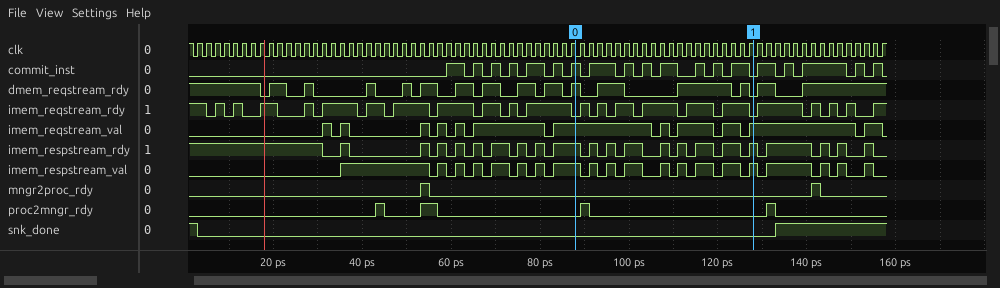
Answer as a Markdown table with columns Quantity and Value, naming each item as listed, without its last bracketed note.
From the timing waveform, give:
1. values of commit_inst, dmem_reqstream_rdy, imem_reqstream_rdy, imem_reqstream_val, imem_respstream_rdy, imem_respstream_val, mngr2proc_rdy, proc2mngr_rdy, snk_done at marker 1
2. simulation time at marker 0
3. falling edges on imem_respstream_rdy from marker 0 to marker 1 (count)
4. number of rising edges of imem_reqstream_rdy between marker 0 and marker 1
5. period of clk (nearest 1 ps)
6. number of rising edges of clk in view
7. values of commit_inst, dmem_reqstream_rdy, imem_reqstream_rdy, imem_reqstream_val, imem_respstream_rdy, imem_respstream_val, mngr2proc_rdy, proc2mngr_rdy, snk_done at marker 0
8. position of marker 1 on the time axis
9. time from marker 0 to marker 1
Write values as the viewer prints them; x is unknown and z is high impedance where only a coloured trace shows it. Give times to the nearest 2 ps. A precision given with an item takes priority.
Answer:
| Quantity | Value |
|---|---|
| values of commit_inst, dmem_reqstream_rdy, imem_reqstream_rdy, imem_reqstream_val, imem_respstream_rdy, imem_respstream_val, mngr2proc_rdy, proc2mngr_rdy, snk_done at marker 1 | commit_inst=0, dmem_reqstream_rdy=0, imem_reqstream_rdy=0, imem_reqstream_val=1, imem_respstream_rdy=1, imem_respstream_val=1, mngr2proc_rdy=0, proc2mngr_rdy=0, snk_done=0 |
| simulation time at marker 0 | 88 ps |
| falling edges on imem_respstream_rdy from marker 0 to marker 1 | 8 |
| number of rising edges of imem_reqstream_rdy between marker 0 and marker 1 | 6 |
| period of clk | 2 ps |
| number of rising edges of clk in view | 78 |
| values of commit_inst, dmem_reqstream_rdy, imem_reqstream_rdy, imem_reqstream_val, imem_respstream_rdy, imem_respstream_val, mngr2proc_rdy, proc2mngr_rdy, snk_done at marker 0 | commit_inst=1, dmem_reqstream_rdy=1, imem_reqstream_rdy=0, imem_reqstream_val=1, imem_respstream_rdy=1, imem_respstream_val=1, mngr2proc_rdy=0, proc2mngr_rdy=0, snk_done=0 |
| position of marker 1 on the time axis | 128 ps |
| time from marker 0 to marker 1 | 40 ps |
